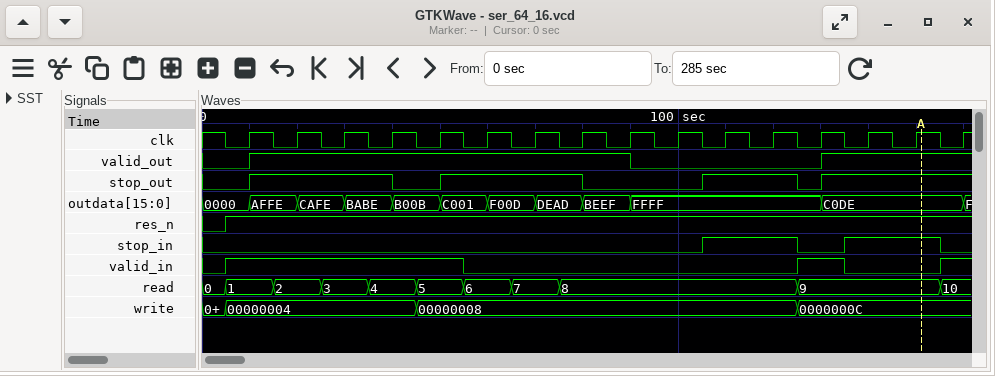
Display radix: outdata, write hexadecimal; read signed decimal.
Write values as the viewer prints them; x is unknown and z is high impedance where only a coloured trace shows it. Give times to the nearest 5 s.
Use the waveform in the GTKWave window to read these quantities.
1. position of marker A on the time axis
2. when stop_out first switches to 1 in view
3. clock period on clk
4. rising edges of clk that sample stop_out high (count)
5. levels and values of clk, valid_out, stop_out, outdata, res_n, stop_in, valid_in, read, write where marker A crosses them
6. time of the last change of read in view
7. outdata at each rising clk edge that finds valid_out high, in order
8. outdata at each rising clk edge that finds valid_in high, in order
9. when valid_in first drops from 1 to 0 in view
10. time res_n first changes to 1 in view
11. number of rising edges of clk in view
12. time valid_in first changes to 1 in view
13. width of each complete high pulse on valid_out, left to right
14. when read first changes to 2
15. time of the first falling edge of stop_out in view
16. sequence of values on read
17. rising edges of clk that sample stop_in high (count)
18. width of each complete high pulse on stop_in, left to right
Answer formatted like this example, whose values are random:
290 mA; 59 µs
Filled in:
150 s; 10 s; 10 s; 11; clk=1, valid_out=1, stop_out=1, outdata=C0DE, res_n=1, stop_in=1, valid_in=0, read=9, write=0000000C; 155 s; AFFE, CAFE, BABE, B00B, C001, F00D, DEAD, BEEF, C0DE, C0DE, C0DE; 0000, AFFE, CAFE, BABE, B00B, FFFF, C0DE; 55 s; 5 s; 16; 5 s; 80 s; 15 s; 40 s; 0, 1, 2, 3, 4, 5, 6, 7, 8, 9, 10; 4; 20 s, 20 s
